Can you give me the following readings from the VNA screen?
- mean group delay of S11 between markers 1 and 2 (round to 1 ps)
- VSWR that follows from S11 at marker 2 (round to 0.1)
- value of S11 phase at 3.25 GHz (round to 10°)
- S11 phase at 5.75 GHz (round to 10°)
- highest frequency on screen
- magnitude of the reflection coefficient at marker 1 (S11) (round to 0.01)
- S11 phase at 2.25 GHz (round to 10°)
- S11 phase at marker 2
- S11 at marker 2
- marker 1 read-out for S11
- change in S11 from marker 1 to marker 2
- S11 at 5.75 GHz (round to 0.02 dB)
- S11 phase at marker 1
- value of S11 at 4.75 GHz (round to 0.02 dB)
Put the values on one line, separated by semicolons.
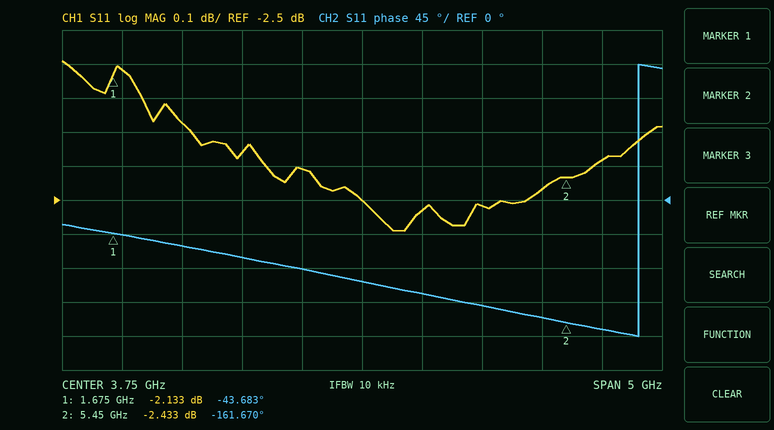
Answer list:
87 ps; 7.2; -90°; -170°; 6.25 GHz; 0.78; -60°; -161.670°; -2.433 dB; -2.133 dB; -0.300 dB; -2.38 dB; -43.683°; -2.52 dB
